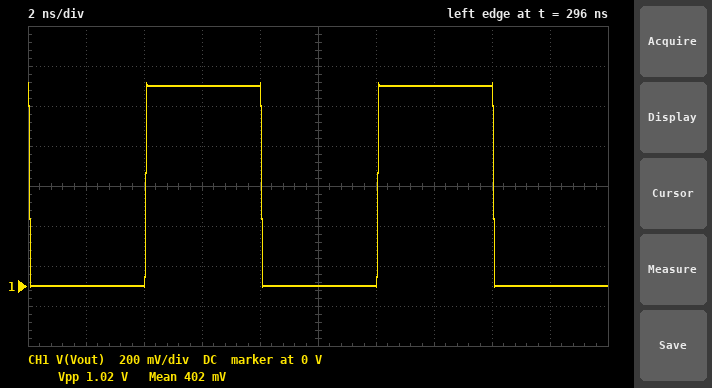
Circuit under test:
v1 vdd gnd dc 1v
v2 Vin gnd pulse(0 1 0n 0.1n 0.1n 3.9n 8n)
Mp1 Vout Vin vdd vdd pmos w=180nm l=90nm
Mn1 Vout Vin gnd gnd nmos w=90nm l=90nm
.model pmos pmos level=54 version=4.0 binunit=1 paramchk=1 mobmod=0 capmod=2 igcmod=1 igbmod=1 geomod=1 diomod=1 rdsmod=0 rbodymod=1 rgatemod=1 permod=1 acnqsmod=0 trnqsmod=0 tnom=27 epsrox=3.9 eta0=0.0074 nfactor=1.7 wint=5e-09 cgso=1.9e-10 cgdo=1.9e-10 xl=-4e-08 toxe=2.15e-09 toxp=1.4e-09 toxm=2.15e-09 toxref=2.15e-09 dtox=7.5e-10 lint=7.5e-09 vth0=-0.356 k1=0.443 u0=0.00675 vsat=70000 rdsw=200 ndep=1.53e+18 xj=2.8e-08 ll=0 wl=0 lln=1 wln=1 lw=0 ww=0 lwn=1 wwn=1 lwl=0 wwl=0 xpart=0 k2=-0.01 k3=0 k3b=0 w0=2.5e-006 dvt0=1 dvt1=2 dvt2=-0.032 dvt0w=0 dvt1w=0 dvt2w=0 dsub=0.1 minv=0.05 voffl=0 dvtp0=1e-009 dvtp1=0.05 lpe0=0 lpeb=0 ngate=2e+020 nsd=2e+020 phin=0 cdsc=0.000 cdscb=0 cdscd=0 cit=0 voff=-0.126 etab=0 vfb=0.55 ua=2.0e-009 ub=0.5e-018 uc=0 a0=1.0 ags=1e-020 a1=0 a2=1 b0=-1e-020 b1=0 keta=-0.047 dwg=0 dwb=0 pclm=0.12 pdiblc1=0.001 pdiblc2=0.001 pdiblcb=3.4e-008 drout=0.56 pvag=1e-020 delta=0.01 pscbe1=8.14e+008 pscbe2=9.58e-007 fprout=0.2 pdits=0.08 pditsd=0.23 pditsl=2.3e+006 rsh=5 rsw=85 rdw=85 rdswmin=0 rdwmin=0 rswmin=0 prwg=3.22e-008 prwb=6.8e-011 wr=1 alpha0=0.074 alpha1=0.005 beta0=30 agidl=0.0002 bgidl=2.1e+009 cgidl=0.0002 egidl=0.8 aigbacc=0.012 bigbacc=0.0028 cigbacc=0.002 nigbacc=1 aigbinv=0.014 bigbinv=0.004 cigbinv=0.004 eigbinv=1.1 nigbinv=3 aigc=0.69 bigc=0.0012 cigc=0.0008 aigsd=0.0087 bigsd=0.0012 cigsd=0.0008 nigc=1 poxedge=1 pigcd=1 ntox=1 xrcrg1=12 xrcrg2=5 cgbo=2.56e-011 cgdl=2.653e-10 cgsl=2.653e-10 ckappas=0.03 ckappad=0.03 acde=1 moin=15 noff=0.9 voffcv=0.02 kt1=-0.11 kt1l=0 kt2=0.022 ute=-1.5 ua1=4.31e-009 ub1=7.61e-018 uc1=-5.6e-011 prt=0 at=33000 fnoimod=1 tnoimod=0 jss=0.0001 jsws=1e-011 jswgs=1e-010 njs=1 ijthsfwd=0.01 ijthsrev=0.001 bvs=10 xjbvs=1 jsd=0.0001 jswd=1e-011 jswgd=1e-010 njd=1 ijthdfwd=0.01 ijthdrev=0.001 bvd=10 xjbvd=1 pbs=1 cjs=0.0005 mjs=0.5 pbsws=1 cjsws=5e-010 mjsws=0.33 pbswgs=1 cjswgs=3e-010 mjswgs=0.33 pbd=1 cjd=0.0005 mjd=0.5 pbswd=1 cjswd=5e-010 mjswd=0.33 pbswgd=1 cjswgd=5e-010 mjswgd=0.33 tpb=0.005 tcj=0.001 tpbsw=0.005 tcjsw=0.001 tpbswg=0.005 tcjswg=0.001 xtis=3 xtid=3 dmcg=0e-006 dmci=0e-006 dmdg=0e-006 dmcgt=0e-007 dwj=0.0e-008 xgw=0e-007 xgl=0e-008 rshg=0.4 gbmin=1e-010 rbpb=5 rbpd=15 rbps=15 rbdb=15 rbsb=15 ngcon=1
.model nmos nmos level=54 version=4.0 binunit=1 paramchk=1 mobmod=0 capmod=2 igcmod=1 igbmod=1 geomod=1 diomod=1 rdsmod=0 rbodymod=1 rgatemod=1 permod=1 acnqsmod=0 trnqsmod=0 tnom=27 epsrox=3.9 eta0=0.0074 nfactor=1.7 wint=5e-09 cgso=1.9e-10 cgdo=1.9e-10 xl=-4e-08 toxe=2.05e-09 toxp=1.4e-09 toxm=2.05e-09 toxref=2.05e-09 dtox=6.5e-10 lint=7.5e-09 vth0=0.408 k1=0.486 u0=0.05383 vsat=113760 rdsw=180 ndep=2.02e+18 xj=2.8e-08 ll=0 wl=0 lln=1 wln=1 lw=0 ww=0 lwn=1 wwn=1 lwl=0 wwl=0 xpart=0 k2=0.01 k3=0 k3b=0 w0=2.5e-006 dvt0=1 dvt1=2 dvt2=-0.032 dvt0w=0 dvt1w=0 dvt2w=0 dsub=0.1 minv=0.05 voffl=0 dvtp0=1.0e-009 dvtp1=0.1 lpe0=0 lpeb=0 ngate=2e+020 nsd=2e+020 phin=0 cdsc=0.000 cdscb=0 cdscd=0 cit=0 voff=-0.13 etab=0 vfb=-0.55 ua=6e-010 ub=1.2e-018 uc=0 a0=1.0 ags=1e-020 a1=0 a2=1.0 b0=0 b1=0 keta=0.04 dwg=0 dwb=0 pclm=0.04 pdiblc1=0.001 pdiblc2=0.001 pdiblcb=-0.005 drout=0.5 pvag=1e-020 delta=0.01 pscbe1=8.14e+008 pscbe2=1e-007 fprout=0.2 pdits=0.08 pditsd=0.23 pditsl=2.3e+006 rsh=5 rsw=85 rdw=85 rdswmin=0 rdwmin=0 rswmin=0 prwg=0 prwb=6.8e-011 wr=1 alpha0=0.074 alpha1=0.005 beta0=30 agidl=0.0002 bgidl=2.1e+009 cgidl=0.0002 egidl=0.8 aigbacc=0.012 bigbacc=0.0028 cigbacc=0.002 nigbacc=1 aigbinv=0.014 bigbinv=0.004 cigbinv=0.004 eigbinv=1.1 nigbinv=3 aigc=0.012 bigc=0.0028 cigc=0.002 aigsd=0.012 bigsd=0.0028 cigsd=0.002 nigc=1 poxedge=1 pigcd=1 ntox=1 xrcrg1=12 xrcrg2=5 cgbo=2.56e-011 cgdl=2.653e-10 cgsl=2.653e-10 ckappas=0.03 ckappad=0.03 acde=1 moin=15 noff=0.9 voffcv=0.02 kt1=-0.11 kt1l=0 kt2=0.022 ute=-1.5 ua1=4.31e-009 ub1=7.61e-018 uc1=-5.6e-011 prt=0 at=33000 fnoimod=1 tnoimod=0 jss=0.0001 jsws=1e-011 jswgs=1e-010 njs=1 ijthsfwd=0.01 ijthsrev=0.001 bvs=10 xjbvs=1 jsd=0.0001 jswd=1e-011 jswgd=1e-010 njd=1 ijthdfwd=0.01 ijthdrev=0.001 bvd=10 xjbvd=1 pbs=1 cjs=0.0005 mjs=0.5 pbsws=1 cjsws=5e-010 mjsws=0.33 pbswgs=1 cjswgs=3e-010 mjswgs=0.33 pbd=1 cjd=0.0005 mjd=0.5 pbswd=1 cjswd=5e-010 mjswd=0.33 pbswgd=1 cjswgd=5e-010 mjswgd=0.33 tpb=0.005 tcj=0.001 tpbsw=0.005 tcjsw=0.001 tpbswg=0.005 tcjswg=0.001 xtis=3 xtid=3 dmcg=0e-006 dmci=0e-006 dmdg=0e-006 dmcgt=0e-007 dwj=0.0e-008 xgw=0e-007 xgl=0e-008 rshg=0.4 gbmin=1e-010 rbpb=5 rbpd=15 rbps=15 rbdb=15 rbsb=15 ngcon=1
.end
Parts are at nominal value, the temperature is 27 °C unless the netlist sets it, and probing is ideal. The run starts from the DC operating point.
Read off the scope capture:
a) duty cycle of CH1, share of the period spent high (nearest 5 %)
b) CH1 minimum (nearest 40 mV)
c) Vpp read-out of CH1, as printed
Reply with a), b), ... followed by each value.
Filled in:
a) 50 %
b) 0 V
c) 1.02 V
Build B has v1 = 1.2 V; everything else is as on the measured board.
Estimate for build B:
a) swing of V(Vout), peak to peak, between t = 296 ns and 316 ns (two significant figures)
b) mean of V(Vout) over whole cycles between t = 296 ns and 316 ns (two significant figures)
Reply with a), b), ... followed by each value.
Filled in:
a) 1.2 V
b) 600 mV
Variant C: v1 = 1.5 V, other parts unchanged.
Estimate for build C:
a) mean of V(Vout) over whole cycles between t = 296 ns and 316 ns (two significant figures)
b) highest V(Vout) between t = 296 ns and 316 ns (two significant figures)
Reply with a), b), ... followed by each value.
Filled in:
a) 790 mV
b) 1.5 V
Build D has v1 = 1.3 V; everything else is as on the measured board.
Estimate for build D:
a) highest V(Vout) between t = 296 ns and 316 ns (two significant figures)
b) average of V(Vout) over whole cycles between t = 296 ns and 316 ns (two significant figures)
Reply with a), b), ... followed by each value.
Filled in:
a) 1.3 V
b) 660 mV
